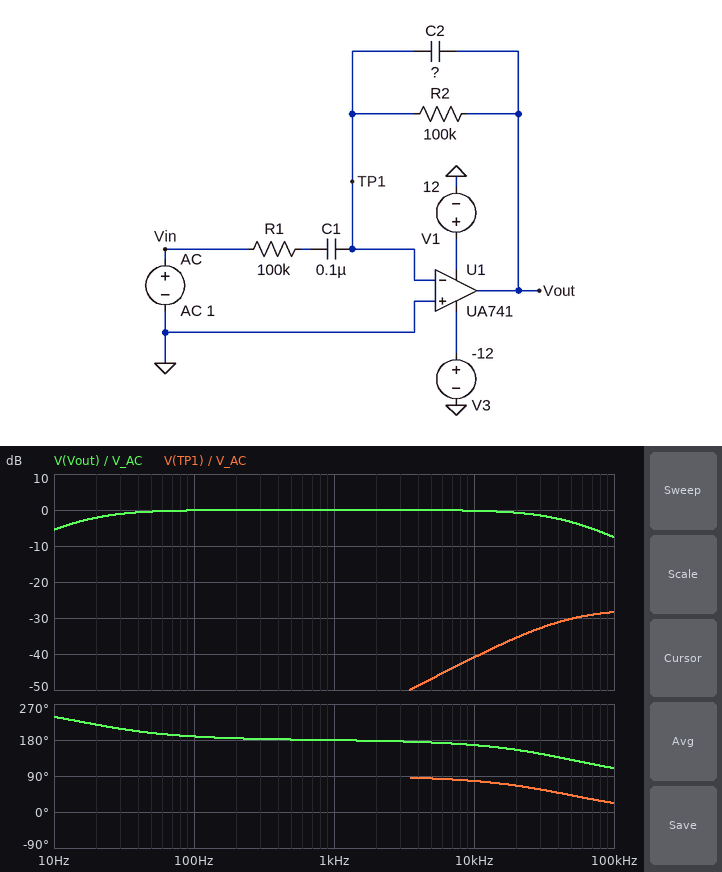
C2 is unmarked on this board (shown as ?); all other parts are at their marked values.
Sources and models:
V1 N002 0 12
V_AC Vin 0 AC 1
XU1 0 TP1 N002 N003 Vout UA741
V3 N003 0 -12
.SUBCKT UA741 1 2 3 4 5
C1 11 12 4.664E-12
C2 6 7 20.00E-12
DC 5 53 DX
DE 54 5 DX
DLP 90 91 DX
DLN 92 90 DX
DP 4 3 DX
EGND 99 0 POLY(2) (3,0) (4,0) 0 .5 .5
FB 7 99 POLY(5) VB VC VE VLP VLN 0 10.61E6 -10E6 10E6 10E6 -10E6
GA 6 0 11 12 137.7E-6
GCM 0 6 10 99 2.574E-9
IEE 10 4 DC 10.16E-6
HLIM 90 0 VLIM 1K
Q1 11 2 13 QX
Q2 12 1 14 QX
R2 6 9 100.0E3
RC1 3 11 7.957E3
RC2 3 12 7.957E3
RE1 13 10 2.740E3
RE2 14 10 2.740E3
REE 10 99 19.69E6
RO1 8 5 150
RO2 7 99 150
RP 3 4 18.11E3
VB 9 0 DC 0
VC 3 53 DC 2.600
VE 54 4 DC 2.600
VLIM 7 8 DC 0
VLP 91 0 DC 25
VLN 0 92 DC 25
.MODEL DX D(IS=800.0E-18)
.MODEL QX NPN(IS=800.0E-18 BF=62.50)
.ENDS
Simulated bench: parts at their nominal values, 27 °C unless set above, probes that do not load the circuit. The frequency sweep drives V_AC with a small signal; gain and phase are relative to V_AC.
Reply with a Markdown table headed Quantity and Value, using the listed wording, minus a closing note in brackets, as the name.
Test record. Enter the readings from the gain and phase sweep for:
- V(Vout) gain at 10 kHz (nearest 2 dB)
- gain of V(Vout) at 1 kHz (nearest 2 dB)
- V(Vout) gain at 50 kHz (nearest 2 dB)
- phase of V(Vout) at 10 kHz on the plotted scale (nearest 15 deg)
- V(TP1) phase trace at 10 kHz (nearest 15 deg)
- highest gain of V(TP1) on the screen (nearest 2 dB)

| Quantity | Value |
|---|---|
| V(Vout) gain at 10 kHz | 0 dB |
| gain of V(Vout) at 1 kHz | 0 dB |
| V(Vout) gain at 50 kHz | -4 dB |
| phase of V(Vout) at 10 kHz on the plotted scale | 165 deg |
| V(TP1) phase trace at 10 kHz | 75 deg |
| highest gain of V(TP1) on the screen | -28 dB |
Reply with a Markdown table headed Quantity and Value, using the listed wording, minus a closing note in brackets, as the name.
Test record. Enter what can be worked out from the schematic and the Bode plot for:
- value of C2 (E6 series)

| Quantity | Value |
|---|---|
| value of C2 | 33 pF |
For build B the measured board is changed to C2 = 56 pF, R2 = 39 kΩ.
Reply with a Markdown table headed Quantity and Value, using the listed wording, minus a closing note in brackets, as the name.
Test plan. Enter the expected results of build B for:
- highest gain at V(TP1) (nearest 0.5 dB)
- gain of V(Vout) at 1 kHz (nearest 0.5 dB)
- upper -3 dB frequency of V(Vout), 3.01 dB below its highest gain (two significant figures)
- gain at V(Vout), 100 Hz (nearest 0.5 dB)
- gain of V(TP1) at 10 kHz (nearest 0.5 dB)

| Quantity | Value |
|---|---|
| highest gain at V(TP1) | -31.5 dB |
| gain of V(Vout) at 1 kHz | -8.0 dB |
| upper -3 dB frequency of V(Vout), 3.01 dB below its highest gain | 71 kHz |
| gain at V(Vout), 100 Hz | -8.5 dB |
| gain of V(TP1) at 10 kHz | -49.0 dB |
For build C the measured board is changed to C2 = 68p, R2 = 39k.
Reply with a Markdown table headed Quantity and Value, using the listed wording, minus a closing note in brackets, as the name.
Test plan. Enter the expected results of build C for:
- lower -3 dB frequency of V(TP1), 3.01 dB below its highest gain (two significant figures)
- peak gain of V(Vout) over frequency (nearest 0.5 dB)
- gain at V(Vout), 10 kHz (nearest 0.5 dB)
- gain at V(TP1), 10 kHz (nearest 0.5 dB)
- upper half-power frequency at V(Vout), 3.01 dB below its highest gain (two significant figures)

| Quantity | Value |
|---|---|
| lower -3 dB frequency of V(TP1), 3.01 dB below its highest gain | 63 kHz |
| peak gain of V(Vout) over frequency | -8.0 dB |
| gain at V(Vout), 10 kHz | -8.5 dB |
| gain at V(TP1), 10 kHz | -49.0 dB |
| upper half-power frequency at V(Vout), 3.01 dB below its highest gain | 59 kHz |
